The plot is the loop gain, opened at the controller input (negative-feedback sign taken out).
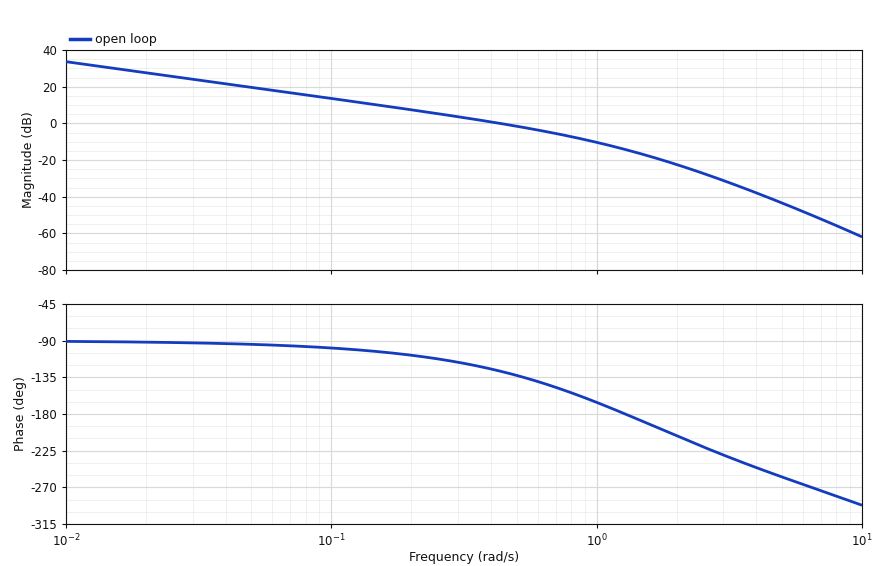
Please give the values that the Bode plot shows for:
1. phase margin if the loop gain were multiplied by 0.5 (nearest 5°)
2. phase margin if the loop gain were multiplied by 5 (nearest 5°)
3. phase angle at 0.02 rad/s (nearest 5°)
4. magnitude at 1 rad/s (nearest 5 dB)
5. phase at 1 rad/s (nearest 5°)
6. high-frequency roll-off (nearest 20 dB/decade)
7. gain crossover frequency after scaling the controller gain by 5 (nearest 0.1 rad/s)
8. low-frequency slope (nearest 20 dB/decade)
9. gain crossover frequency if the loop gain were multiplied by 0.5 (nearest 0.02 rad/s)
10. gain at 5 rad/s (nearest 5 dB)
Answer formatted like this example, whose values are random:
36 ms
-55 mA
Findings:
70°
0°
-90°
-10 dB
-165°
-60 dB/decade
1.3 rad/s
-20 dB/decade
0.24 rad/s
-45 dB
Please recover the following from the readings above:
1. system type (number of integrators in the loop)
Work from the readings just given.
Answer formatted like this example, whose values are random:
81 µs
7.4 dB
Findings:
1
